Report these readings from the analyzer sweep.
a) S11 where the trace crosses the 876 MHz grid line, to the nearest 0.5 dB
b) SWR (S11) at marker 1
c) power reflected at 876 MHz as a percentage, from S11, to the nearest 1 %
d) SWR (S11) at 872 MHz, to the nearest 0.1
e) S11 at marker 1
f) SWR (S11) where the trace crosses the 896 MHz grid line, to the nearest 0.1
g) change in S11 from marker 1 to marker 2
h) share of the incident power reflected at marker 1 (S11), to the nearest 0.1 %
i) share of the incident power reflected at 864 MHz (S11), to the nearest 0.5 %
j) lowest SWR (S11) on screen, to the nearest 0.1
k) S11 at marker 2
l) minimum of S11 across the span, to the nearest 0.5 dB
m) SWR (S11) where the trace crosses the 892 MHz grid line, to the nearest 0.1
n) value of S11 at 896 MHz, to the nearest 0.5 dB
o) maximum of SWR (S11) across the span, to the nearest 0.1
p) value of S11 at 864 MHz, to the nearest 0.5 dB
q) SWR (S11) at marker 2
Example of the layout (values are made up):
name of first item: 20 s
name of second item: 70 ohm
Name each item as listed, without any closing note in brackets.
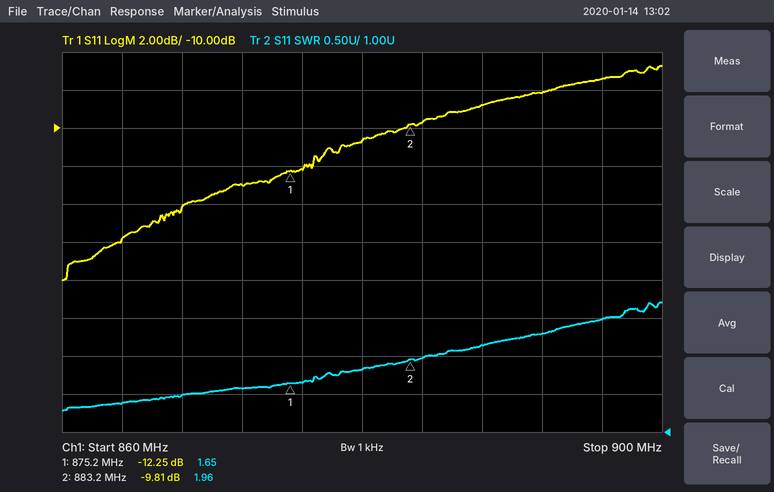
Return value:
S11 where the trace crosses the 876 MHz grid line, to the nearest 0.5 dB: -12.0 dB
SWR (S11) at marker 1: 1.65
power reflected at 876 MHz as a percentage, from S11, to the nearest 1 %: 6 %
SWR (S11) at 872 MHz, to the nearest 0.1: 1.6
S11 at marker 1: -12.25 dB
SWR (S11) where the trace crosses the 896 MHz grid line, to the nearest 0.1: 2.5
change in S11 from marker 1 to marker 2: 2.44 dB
share of the incident power reflected at marker 1 (S11), to the nearest 0.1 %: 6.0 %
share of the incident power reflected at 864 MHz (S11), to the nearest 0.5 %: 2.5 %
lowest SWR (S11) on screen, to the nearest 0.1: 1.3
S11 at marker 2: -9.81 dB
minimum of S11 across the span, to the nearest 0.5 dB: -18.0 dB
SWR (S11) where the trace crosses the 892 MHz grid line, to the nearest 0.1: 2.3
value of S11 at 896 MHz, to the nearest 0.5 dB: -7.5 dB
maximum of SWR (S11) across the span, to the nearest 0.1: 2.7
value of S11 at 864 MHz, to the nearest 0.5 dB: -16.0 dB
SWR (S11) at marker 2: 1.96
